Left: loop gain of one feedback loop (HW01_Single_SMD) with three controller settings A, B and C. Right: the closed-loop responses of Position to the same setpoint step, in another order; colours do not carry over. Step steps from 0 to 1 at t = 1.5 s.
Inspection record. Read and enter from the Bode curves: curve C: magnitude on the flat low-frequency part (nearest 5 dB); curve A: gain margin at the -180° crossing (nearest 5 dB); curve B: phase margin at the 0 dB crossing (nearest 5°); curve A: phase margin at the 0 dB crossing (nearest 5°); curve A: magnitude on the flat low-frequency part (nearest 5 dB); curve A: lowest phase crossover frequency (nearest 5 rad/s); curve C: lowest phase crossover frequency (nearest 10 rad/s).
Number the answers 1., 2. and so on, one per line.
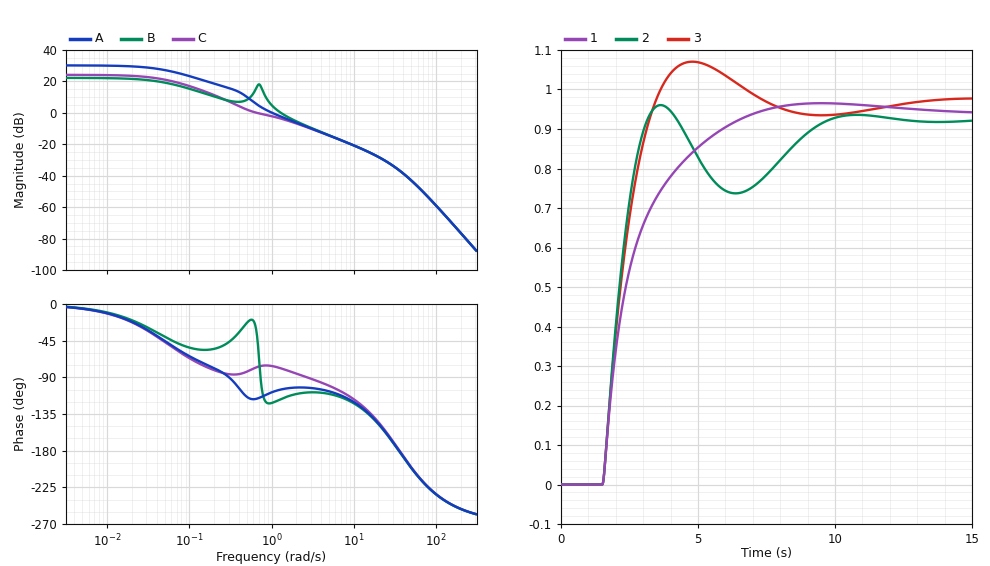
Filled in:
1. 25 dB
2. 35 dB
3. 65°
4. 70°
5. 30 dB
6. 35 rad/s
7. 40 rad/s
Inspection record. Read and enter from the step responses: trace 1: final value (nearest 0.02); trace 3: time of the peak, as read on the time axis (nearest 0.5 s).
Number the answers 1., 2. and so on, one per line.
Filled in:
1. 0.94
2. 5.0 s
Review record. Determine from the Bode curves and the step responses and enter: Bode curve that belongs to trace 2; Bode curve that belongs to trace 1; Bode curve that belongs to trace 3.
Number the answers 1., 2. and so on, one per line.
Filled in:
1. B
2. C
3. A
